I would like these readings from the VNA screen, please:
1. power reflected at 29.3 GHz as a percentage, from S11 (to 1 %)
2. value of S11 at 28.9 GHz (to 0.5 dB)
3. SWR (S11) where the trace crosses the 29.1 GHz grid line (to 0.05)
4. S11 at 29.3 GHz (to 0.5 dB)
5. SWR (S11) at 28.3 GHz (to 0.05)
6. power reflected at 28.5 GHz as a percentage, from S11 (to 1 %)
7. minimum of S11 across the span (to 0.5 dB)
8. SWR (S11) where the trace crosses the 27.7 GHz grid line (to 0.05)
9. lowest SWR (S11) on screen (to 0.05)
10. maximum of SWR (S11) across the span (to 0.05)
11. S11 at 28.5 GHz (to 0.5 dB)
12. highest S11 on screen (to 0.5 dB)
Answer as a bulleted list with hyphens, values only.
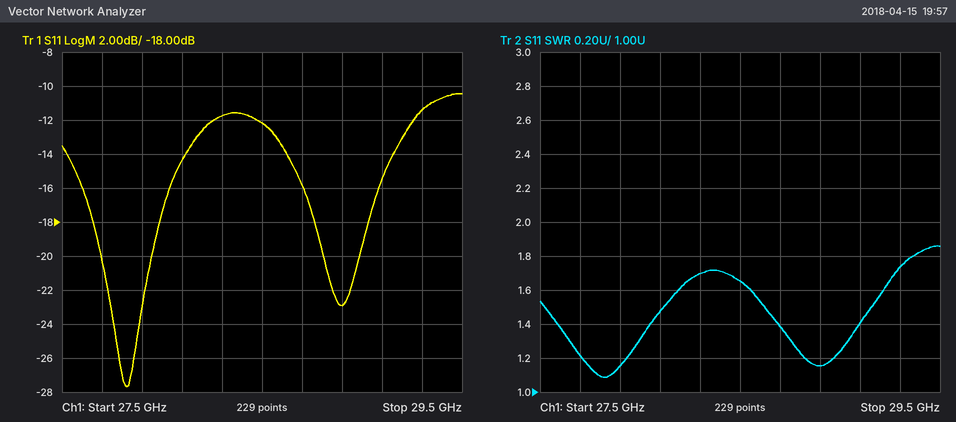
- 7 %
- -23.0 dB
- 1.40
- -11.5 dB
- 1.70
- 6 %
- -27.5 dB
- 1.20
- 1.10
- 1.85
- -12.0 dB
- -10.5 dB
